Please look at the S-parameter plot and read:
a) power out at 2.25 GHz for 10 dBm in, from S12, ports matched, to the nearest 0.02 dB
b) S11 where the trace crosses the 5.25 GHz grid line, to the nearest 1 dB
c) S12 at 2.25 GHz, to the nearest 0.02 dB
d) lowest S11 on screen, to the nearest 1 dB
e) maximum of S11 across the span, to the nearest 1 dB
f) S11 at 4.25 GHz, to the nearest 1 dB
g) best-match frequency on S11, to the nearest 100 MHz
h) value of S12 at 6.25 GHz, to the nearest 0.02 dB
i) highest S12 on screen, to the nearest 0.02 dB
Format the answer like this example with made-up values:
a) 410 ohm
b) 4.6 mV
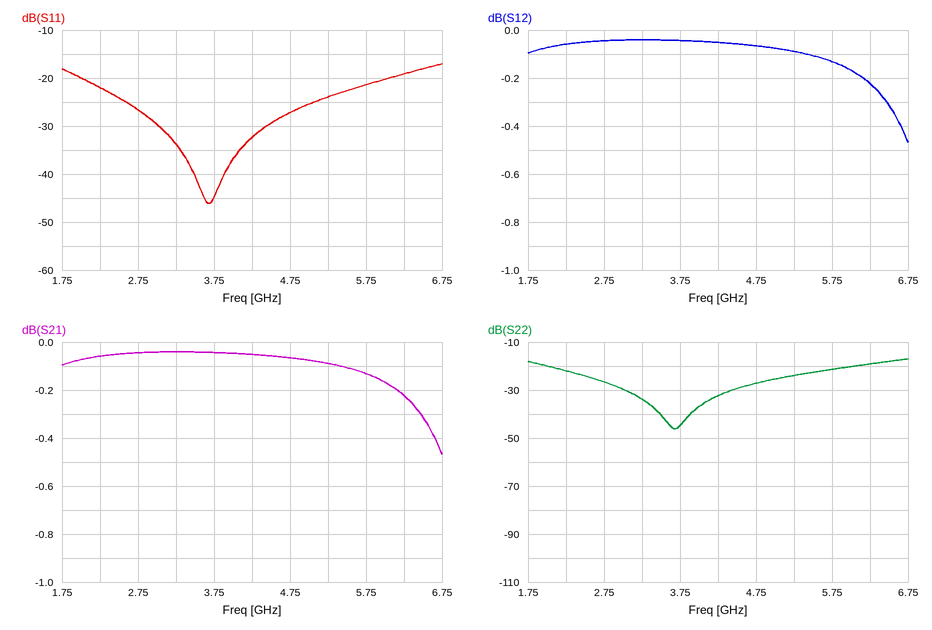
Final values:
a) 9.94 dBm
b) -24 dB
c) -0.06 dB
d) -46 dB
e) -17 dB
f) -32 dB
g) 3.7 GHz
h) -0.22 dB
i) -0.04 dB
